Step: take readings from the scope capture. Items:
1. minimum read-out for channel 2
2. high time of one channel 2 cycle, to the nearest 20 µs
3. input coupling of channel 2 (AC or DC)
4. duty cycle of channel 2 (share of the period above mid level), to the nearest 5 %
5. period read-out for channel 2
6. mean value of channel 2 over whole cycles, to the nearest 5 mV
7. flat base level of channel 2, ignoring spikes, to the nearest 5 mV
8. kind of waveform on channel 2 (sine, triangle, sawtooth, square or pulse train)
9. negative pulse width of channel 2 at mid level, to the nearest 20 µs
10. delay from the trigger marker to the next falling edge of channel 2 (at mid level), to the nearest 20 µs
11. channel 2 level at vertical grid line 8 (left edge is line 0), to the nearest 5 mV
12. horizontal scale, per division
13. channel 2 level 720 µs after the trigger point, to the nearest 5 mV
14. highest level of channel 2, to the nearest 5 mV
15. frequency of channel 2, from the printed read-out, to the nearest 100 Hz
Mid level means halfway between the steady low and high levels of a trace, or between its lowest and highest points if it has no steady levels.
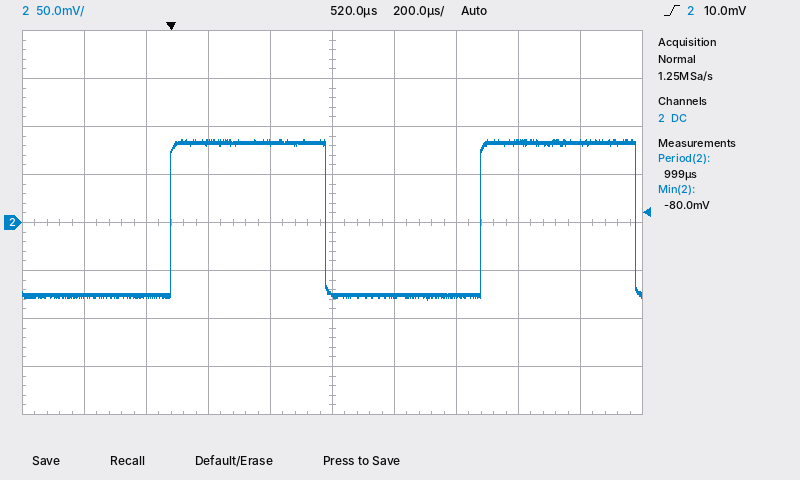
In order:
-80.0 mV
500 µs
DC
50 %
999 µs
5 mV
-75 mV
square
500 µs
500 µs
85 mV
200 µs
-75 mV
85 mV
1.0 kHz
